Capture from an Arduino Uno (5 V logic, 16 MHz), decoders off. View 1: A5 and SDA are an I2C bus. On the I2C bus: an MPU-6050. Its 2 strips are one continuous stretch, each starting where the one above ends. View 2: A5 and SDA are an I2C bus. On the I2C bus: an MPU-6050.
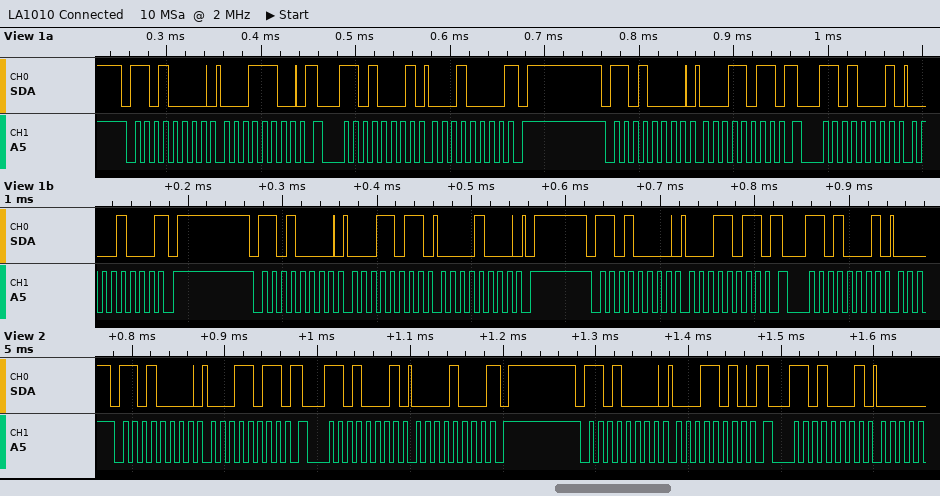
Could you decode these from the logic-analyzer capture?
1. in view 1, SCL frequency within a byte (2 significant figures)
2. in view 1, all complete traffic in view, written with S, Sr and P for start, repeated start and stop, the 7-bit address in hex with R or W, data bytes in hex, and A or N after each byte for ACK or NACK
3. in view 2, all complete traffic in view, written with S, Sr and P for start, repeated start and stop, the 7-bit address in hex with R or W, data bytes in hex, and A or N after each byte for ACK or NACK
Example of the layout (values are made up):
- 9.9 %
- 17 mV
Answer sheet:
- 100 kHz
- S 68W A 1C A Sr 68R A 10 N P S 68W A 1B A Sr 68R A 08 N P S 68W A 1B A 08 A P S 68W A 1B A Sr 68R A
- S 68W A 1B A Sr 68R A 08 N P S 68W A 1A A Sr 68R A
